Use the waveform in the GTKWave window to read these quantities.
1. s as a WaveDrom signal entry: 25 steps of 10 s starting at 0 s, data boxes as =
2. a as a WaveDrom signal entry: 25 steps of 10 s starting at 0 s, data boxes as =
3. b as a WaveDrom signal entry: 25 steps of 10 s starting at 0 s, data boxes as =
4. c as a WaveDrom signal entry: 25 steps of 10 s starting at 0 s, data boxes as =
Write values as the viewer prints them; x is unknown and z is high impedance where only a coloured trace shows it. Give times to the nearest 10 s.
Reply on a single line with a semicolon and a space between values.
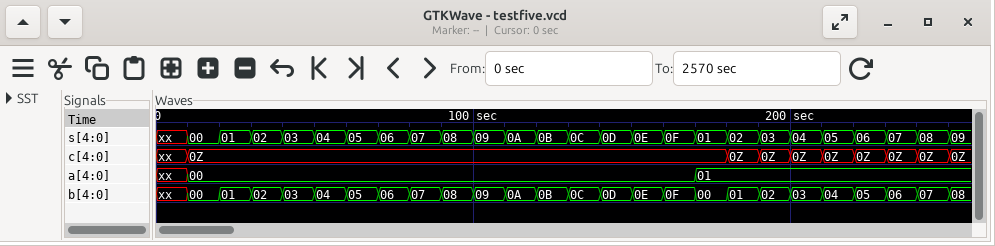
{name: 's', wave: 'x========================', data: '00 01 02 03 04 05 06 07 08 09 0A 0B 0C 0D 0E 0F 01 02 03 04 05 06 07 08'}; {name: 'a', wave: 'x=...............=.......', data: '00 01'}; {name: 'b', wave: 'x========================', data: '00 01 02 03 04 05 06 07 08 09 0A 0B 0C 0D 0E 0F 00 01 02 03 04 05 06 07'}; {name: 'c', wave: '==................=======', data: 'xx 0Z 0Z 0Z 0Z 0Z 0Z 0Z 0Z'}
